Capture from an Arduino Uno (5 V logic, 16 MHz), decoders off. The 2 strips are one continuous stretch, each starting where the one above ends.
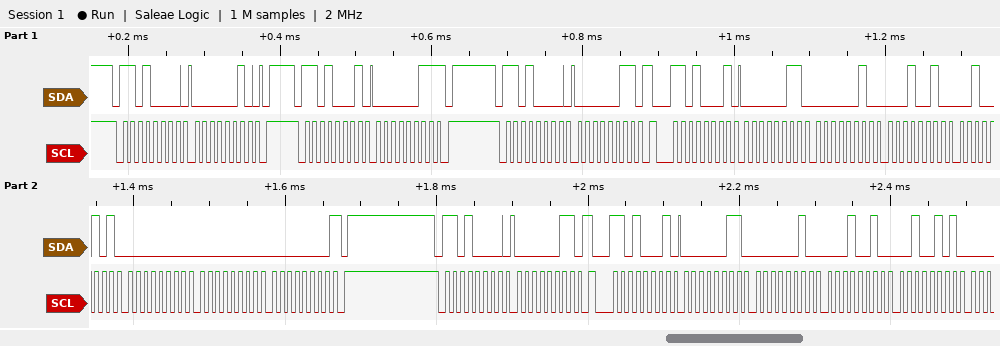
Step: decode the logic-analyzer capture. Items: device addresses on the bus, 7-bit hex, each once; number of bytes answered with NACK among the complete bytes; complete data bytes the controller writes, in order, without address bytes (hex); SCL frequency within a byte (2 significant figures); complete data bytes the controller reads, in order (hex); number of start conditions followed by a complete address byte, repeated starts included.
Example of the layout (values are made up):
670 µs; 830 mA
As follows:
0x68; 2; 02 03 03; 100 kHz; 03 03 02 12 25 00 00 00 03 02 12 25; 6
